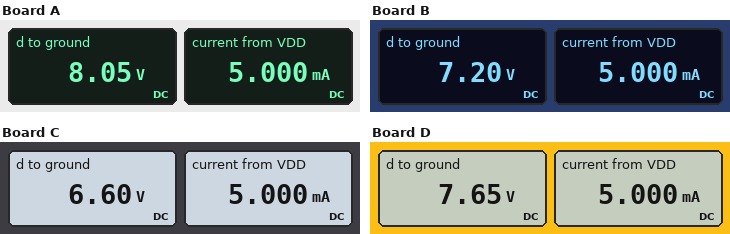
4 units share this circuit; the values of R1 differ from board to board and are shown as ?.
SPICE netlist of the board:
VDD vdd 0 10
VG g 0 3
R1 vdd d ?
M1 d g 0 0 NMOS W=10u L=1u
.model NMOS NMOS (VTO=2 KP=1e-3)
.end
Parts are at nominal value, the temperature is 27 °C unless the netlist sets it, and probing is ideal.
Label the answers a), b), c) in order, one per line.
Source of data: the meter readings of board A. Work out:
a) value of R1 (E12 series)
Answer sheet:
a) 390 Ω
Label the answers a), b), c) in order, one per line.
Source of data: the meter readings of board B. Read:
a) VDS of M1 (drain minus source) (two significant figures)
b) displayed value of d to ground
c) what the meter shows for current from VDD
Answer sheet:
a) 7.2 V
b) 7.20 V
c) 5.000 mA
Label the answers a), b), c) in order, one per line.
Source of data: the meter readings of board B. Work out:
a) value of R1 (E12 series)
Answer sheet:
a) 560 Ω
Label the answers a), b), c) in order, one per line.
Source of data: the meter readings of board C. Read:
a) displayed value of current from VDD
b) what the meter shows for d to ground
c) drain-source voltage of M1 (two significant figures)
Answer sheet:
a) 5.000 mA
b) 6.60 V
c) 6.6 V
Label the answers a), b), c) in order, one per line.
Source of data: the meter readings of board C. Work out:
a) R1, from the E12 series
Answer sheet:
a) 680 Ω
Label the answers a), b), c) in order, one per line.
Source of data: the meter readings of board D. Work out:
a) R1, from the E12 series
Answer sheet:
a) 470 Ω
